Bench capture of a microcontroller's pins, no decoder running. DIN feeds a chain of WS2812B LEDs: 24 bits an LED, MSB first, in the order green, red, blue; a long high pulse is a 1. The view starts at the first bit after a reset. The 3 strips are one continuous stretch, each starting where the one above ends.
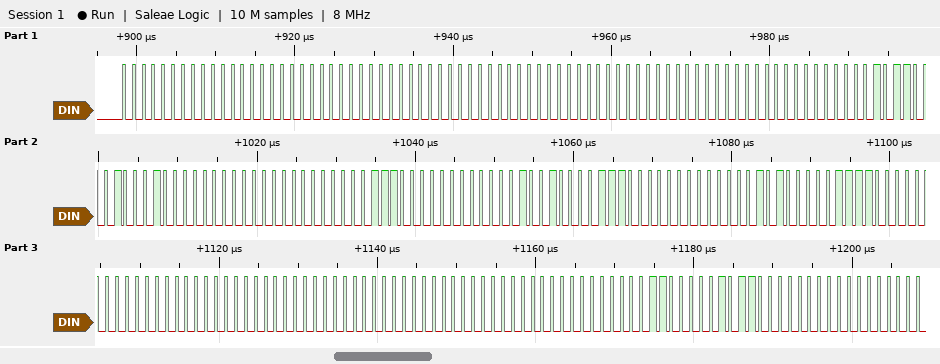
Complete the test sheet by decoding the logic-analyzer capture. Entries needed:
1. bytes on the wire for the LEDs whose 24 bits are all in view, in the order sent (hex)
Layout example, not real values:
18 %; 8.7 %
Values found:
00 00 00 00 00 00 00 00 00 0B 11 00 00 07 00 09 0E 00 0A 0F 00 00 00 00 00 00 00 06 0B 00
